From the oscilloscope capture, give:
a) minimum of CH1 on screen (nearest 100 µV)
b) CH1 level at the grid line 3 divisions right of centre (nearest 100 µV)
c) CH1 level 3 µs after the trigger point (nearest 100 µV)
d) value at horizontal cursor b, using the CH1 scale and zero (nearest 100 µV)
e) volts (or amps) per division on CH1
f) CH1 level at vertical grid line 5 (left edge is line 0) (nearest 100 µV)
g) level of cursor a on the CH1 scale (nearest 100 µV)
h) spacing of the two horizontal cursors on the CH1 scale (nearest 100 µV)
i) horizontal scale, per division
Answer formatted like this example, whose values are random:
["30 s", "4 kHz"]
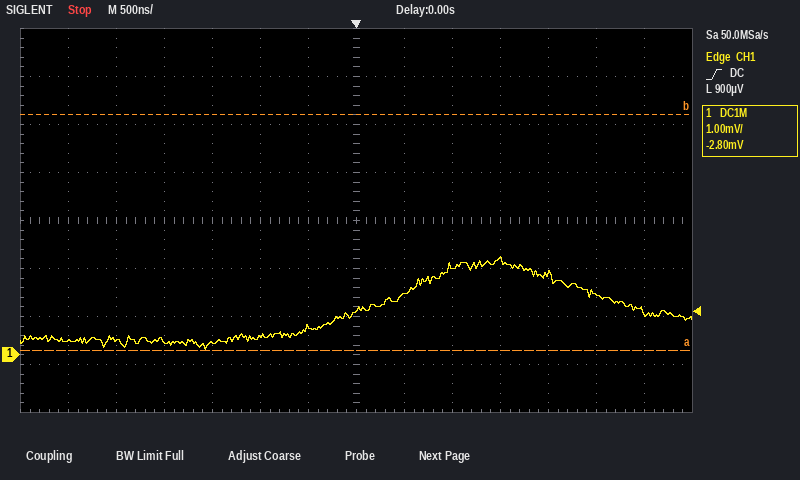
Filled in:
["100 µV", "2.0 mV", "900 µV", "5.0 mV", "1 mV", "400 µV", "100 µV", "4.9 mV", "500 ns"]
